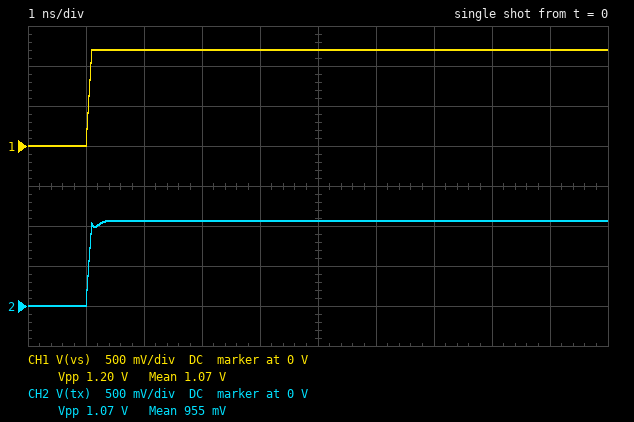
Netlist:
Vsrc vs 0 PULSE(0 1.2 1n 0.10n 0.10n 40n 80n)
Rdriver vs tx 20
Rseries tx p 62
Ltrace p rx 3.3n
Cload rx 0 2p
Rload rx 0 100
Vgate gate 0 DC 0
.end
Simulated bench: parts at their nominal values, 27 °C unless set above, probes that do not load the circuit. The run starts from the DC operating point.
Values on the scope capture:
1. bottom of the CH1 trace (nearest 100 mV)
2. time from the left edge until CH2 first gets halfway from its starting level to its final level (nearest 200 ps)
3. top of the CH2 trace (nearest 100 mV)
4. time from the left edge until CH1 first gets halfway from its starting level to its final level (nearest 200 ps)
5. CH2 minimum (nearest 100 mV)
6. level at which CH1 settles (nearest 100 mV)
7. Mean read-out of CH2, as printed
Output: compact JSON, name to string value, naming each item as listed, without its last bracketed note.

{"bottom of the CH1 trace": "0 V", "time from the left edge until CH2 first gets halfway from its starting level to its final level": "1.0 ns", "top of the CH2 trace": "1.1 V", "time from the left edge until CH1 first gets halfway from its starting level to its final level": "1.0 ns", "CH2 minimum": "0 V", "level at which CH1 settles": "1.2 V", "Mean read-out of CH2, as printed": "955 mV"}
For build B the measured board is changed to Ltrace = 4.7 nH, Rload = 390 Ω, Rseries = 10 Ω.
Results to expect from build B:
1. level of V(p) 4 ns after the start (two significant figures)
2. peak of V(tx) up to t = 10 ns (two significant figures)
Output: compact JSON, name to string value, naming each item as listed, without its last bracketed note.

{"level of V(p) 4 ns after the start": "1.1 V", "peak of V(tx) up to t = 10 ns": "1.2 V"}
